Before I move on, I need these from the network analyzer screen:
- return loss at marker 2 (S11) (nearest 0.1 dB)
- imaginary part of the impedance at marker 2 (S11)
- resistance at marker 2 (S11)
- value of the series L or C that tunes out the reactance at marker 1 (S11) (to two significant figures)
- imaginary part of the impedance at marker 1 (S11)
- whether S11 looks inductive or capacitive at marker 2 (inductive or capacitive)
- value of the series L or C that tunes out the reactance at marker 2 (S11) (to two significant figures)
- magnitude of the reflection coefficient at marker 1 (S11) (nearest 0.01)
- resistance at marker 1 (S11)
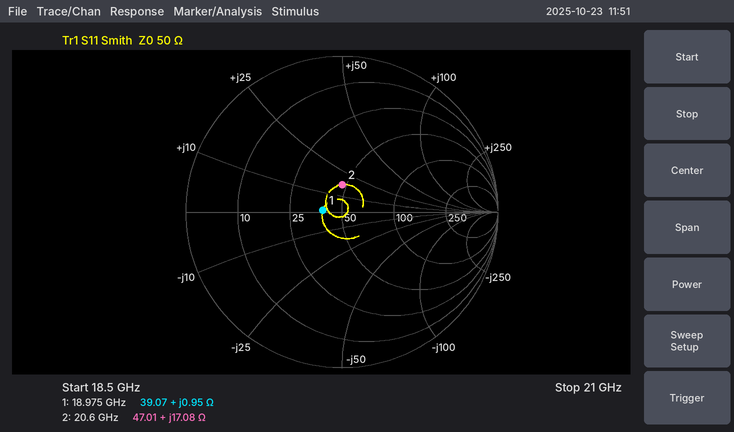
15.1 dB
+17.08 Ω
47.01 Ω
8.8 pF
+0.95 Ω
inductive
450 fF
0.12
39.07 Ω
